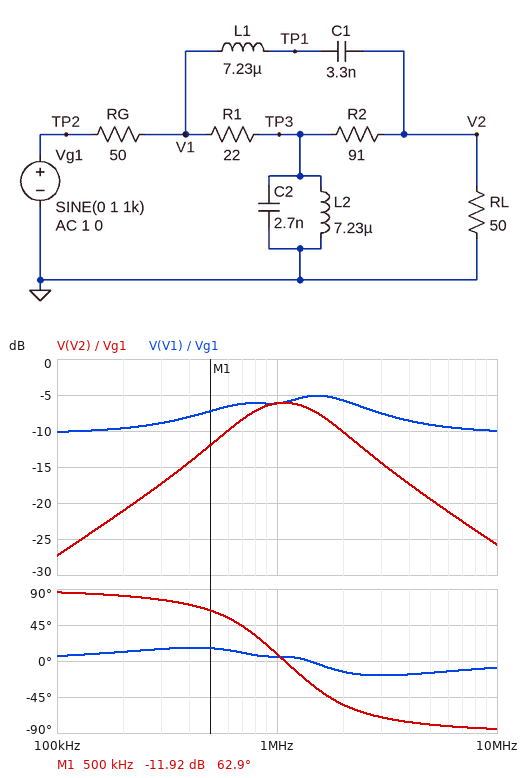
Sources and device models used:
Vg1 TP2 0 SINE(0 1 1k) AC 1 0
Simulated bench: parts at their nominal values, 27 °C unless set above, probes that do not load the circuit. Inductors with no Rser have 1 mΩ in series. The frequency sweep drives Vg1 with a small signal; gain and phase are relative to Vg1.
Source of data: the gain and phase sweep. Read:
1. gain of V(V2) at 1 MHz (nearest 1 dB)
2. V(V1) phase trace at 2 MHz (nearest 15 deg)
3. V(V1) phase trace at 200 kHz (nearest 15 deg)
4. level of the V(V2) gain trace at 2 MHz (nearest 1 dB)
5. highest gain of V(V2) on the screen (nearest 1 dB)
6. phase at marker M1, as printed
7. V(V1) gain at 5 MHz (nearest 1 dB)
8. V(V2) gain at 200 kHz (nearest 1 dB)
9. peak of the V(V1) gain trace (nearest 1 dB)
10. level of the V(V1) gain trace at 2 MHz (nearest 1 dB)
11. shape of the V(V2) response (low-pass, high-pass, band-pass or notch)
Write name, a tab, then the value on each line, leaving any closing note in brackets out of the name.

gain of V(V2) at 1 MHz	-6 dB
V(V1) phase trace at 2 MHz	-15 deg
V(V1) phase trace at 200 kHz	15 deg
level of the V(V2) gain trace at 2 MHz	-10 dB
highest gain of V(V2) on the screen	-6 dB
phase at marker M1, as printed	62.9 deg
V(V1) gain at 5 MHz	-9 dB
V(V2) gain at 200 kHz	-21 dB
peak of the V(V1) gain trace	-5 dB
level of the V(V1) gain trace at 2 MHz	-6 dB
shape of the V(V2) response	band-pass
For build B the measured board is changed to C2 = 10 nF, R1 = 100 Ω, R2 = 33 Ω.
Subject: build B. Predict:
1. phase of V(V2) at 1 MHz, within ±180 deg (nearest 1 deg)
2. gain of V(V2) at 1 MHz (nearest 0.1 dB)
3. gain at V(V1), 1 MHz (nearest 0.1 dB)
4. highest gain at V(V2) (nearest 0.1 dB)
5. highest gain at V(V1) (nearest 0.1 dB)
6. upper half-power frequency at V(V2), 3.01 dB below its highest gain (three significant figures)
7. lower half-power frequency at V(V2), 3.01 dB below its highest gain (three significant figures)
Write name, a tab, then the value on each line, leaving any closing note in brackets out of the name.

phase of V(V2) at 1 MHz, within ±180 deg	-16 deg
gain of V(V2) at 1 MHz	-10.2 dB
gain at V(V1), 1 MHz	-9.8 dB
highest gain at V(V2)	-8.2 dB
highest gain at V(V1)	-3.5 dB
upper half-power frequency at V(V2), 3.01 dB below its highest gain	1.33 MHz
lower half-power frequency at V(V2), 3.01 dB below its highest gain	436 kHz
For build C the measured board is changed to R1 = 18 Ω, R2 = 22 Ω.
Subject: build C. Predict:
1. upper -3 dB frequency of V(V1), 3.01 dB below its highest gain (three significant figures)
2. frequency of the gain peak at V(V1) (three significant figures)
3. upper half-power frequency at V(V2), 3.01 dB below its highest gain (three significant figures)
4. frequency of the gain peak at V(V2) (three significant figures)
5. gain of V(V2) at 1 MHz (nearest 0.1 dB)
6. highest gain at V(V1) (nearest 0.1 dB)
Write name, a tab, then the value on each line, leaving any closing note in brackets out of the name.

upper -3 dB frequency of V(V1), 3.01 dB below its highest gain	3.19 MHz
frequency of the gain peak at V(V1)	1.42 MHz
upper half-power frequency at V(V2), 3.01 dB below its highest gain	1.85 MHz
frequency of the gain peak at V(V2)	1.05 MHz
gain of V(V2) at 1 MHz	-6.1 dB
highest gain at V(V1)	-5.2 dB
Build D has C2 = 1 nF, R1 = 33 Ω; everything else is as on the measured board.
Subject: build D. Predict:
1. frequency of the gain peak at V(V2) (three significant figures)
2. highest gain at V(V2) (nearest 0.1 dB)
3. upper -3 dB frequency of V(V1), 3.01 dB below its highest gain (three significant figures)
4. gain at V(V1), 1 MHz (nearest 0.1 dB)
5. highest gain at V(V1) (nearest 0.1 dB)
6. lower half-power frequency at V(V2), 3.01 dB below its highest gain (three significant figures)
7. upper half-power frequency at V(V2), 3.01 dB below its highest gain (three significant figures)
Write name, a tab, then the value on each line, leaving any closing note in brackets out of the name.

frequency of the gain peak at V(V2)	1.11 MHz
highest gain at V(V2)	-7.3 dB
upper -3 dB frequency of V(V1), 3.01 dB below its highest gain	6.79 MHz
gain at V(V1), 1 MHz	-7.5 dB
highest gain at V(V1)	-3.2 dB
lower half-power frequency at V(V2), 3.01 dB below its highest gain	615 kHz
upper half-power frequency at V(V2), 3.01 dB below its highest gain	2.80 MHz
